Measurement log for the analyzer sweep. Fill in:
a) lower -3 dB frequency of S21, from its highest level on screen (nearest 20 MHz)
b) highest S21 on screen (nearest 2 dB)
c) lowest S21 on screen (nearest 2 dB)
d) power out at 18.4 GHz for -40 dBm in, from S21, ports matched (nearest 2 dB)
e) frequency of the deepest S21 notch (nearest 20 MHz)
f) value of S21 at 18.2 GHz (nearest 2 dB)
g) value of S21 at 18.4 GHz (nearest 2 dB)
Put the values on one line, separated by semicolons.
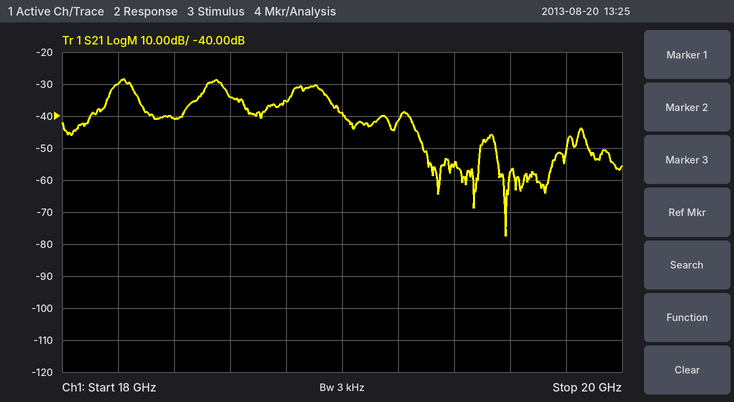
18.18 GHz; -28 dB; -78 dB; -80 dBm; 19.58 GHz; -30 dB; -40 dB
